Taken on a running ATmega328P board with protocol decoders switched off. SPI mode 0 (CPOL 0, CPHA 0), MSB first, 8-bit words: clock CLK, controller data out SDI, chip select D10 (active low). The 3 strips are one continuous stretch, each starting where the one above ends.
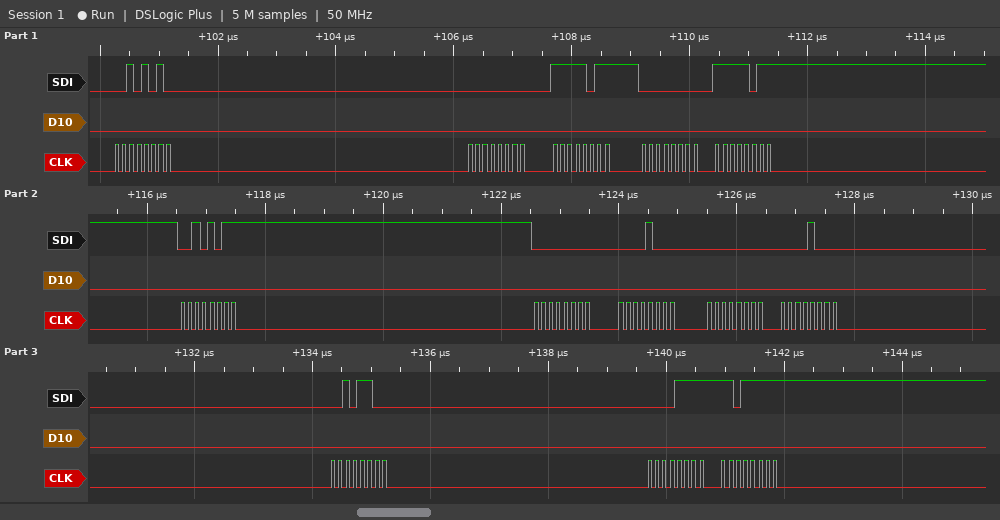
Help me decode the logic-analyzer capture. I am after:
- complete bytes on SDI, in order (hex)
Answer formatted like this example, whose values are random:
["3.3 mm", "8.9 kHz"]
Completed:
["2A 00 FB 00 FB 2B 00 08 00 08 2C 0F DF"]
